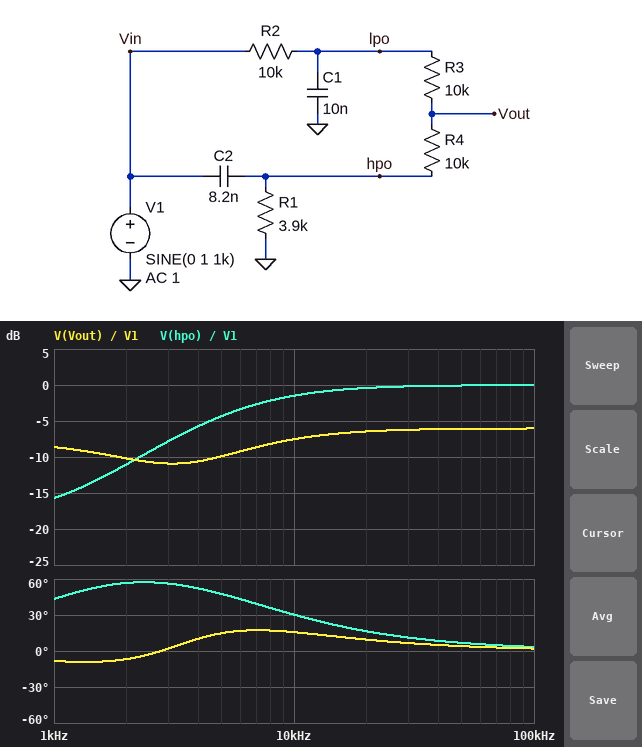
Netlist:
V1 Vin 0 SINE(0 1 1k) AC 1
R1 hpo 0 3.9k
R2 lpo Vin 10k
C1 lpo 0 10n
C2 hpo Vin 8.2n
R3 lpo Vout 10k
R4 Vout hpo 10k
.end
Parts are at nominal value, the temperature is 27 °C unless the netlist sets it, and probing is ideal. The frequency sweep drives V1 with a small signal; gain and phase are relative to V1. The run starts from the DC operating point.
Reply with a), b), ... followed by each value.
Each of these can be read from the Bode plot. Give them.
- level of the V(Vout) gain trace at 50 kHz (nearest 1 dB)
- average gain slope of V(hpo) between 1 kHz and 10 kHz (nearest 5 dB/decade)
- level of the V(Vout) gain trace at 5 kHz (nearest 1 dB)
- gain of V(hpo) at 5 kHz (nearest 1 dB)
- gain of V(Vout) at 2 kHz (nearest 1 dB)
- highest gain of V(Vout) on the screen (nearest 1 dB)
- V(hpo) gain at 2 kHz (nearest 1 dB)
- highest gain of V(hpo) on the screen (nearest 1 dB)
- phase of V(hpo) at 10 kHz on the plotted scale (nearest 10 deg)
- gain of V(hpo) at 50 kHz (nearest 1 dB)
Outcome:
a) -6 dB
b) 15 dB/decade
c) -10 dB
d) -4 dB
e) -10 dB
f) -6 dB
g) -11 dB
h) 0 dB
i) 30 deg
j) 0 dB
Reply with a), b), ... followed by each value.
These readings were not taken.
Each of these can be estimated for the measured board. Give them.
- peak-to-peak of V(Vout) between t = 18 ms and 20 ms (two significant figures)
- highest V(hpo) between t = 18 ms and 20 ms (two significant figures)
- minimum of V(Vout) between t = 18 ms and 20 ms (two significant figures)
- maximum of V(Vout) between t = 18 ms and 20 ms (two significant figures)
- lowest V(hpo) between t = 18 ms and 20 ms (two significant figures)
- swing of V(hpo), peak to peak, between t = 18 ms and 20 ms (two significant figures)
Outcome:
a) 740 mV
b) 160 mV
c) -370 mV
d) 370 mV
e) -160 mV
f) 330 mV
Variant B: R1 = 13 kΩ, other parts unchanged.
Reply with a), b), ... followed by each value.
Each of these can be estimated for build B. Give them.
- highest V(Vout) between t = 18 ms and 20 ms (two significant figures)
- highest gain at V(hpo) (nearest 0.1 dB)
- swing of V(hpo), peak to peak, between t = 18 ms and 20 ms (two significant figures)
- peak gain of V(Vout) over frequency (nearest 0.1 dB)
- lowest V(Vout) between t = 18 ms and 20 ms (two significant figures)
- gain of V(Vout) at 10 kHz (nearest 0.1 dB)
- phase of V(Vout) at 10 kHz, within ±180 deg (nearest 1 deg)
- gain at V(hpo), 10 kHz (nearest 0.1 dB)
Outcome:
a) 510 mV
b) 0 dB
c) 770 mV
d) -5.4 dB
e) -510 mV
f) -6.1 dB
g) 0 deg
h) -0.4 dB
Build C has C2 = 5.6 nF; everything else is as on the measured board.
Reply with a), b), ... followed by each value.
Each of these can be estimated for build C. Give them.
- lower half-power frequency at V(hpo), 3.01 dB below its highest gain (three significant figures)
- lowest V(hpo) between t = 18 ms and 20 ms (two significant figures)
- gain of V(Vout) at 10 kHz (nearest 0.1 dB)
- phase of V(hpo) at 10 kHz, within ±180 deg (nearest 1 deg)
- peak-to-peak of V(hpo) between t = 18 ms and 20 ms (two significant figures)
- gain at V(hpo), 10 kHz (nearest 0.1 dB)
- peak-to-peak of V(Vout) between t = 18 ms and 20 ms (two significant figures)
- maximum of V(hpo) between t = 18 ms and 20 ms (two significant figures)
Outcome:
a) 9.26 kHz
b) -120 mV
c) -9.1 dB
d) 40 deg
e) 250 mV
f) -2.7 dB
g) 730 mV
h) 120 mV
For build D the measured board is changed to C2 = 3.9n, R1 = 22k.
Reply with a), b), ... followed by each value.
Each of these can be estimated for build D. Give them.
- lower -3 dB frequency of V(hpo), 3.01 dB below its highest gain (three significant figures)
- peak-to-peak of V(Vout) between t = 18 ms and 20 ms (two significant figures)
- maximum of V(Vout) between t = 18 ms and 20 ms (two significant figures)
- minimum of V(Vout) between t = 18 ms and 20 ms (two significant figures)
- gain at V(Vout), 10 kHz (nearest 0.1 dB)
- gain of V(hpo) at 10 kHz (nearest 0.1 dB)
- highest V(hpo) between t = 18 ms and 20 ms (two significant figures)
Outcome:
a) 5.21 kHz
b) 1.1 V
c) 530 mV
d) -530 mV
e) -6.8 dB
f) -1.0 dB
g) 360 mV
